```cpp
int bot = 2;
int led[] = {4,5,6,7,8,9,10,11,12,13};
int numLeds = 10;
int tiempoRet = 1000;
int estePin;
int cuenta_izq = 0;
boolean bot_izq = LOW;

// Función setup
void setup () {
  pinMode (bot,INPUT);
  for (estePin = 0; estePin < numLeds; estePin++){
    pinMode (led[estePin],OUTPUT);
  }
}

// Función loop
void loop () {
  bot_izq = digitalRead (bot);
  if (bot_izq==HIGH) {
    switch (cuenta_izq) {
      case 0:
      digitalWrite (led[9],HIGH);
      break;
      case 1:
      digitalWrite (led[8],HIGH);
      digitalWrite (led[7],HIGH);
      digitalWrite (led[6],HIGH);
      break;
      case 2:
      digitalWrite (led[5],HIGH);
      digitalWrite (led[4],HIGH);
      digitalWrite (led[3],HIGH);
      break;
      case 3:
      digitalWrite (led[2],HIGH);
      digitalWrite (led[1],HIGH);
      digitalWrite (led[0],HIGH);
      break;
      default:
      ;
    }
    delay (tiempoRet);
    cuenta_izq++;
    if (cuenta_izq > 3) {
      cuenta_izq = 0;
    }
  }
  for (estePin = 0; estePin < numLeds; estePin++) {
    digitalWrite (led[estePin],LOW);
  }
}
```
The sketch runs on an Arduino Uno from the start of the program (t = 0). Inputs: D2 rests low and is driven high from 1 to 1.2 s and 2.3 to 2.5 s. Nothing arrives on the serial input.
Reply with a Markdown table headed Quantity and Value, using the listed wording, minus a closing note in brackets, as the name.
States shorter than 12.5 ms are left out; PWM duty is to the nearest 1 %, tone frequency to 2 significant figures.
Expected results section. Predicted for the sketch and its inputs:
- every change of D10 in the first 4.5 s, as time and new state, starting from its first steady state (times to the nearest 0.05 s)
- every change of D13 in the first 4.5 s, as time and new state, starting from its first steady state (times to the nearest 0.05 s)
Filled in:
| Quantity | Value |
|---|---|
| every change of D10 in the first 4.5 s, as time and new state, starting from its first steady state | 0 s low; 2.3 s high; 3.3 s low |
| every change of D13 in the first 4.5 s, as time and new state, starting from its first steady state | 0 s low; 1 s high; 2 s low |
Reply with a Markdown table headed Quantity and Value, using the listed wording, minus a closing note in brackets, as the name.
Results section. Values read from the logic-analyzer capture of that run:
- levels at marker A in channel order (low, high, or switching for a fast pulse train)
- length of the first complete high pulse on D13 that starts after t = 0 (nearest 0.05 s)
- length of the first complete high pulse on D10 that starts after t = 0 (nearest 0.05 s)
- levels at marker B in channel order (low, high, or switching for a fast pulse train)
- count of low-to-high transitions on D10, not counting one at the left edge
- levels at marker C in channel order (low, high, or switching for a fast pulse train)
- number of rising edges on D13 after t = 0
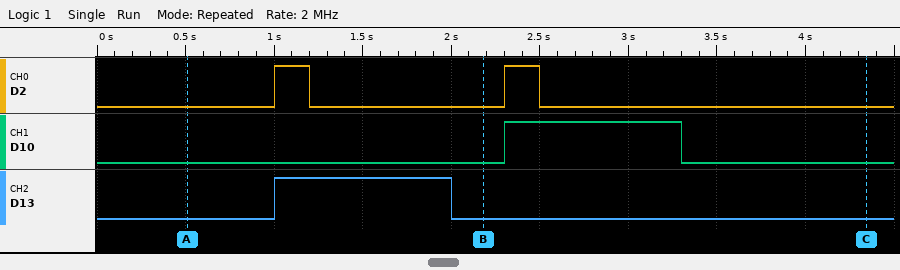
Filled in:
| Quantity | Value |
|---|---|
| levels at marker A in channel order | D2 low, D10 low, D13 low |
| length of the first complete high pulse on D13 that starts after t = 0 | 1.00 s |
| length of the first complete high pulse on D10 that starts after t = 0 | 1.00 s |
| levels at marker B in channel order | D2 low, D10 low, D13 low |
| count of low-to-high transitions on D10, not counting one at the left edge | 1 |
| levels at marker C in channel order | D2 low, D10 low, D13 low |
| number of rising edges on D13 after t = 0 | 1 |
